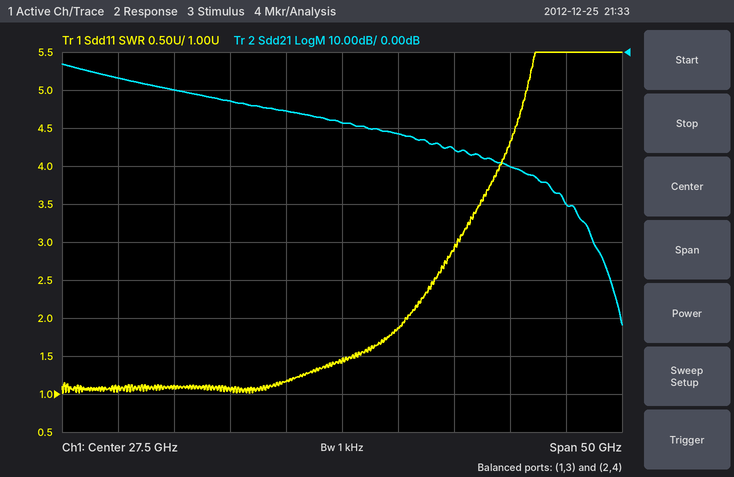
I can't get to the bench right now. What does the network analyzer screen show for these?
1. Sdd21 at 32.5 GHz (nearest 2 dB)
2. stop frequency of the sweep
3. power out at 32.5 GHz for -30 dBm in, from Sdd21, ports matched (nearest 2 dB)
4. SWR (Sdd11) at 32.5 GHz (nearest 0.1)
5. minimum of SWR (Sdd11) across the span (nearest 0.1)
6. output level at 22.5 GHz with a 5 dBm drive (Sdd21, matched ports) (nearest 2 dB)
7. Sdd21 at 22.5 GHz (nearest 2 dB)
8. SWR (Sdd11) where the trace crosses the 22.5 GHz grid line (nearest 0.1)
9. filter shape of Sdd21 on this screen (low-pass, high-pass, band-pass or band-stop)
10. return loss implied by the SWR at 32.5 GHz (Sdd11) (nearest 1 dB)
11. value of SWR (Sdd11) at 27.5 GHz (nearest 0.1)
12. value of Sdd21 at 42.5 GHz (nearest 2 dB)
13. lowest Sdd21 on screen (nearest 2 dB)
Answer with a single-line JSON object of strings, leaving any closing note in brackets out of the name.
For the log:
{"Sdd21 at 32.5 GHz": "-22 dB", "stop frequency of the sweep": "52.5 GHz", "power out at 32.5 GHz for -30 dBm in, from Sdd21, ports matched": "-52 dBm", "SWR (Sdd11) at 32.5 GHz": "1.9", "minimum of SWR (Sdd11) across the span": "1.0", "output level at 22.5 GHz with a 5 dBm drive (Sdd21, matched ports)": "-10 dBm", "Sdd21 at 22.5 GHz": "-16 dB", "SWR (Sdd11) where the trace crosses the 22.5 GHz grid line": "1.2", "filter shape of Sdd21 on this screen": "low-pass", "return loss implied by the SWR at 32.5 GHz (Sdd11)": "10 dB", "value of SWR (Sdd11) at 27.5 GHz": "1.4", "value of Sdd21 at 42.5 GHz": "-30 dB", "lowest Sdd21 on screen": "-72 dB"}
